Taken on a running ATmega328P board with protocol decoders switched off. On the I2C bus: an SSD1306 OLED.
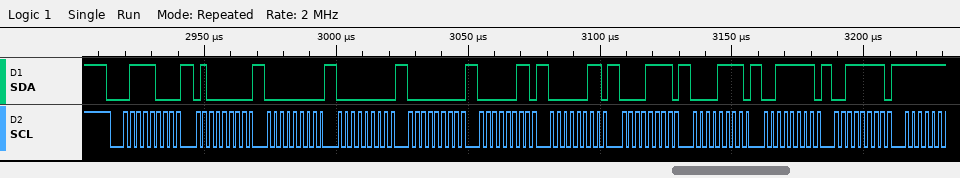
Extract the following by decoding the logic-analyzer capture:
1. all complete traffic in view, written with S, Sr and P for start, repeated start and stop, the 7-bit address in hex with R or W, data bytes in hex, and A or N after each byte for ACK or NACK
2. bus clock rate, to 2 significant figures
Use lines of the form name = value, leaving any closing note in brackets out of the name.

all complete traffic in view, written with S, Sr and P for start, repeated start and stop, the 7-bit address in hex with R or W, data bytes in hex, and A or N after each byte for ACK or NACK = S 3CW A 40 A 00 A 00 A 00 A 03 A 03 A 0F A 0F A 3F A 3F A
bus clock rate, to 2 significant figures = 400 kHz
